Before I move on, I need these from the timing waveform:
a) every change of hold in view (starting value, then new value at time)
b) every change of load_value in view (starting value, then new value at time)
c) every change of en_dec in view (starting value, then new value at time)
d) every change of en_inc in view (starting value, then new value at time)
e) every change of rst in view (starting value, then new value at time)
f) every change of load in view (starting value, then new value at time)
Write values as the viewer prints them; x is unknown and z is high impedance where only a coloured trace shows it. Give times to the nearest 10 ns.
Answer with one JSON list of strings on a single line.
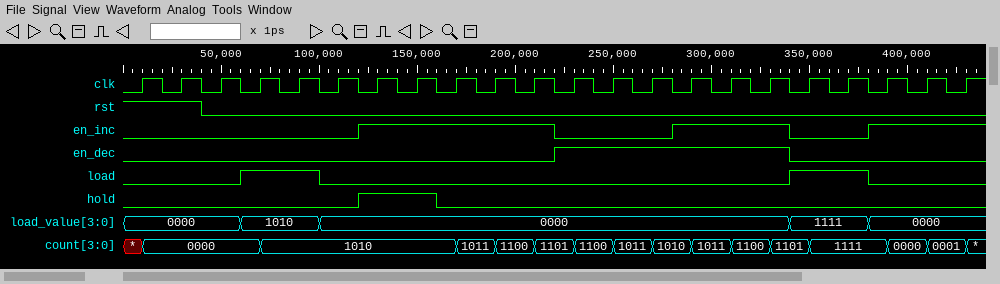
["0, 1 at 120 ns, 0 at 160 ns", "0000, 1010 at 60 ns, 0000 at 100 ns, 1111 at 340 ns, 0000 at 380 ns", "0, 1 at 220 ns, 0 at 340 ns", "0, 1 at 120 ns, 0 at 220 ns, 1 at 280 ns, 0 at 340 ns, 1 at 380 ns", "1, 0 at 40 ns", "0, 1 at 60 ns, 0 at 100 ns, 1 at 340 ns, 0 at 380 ns"]
